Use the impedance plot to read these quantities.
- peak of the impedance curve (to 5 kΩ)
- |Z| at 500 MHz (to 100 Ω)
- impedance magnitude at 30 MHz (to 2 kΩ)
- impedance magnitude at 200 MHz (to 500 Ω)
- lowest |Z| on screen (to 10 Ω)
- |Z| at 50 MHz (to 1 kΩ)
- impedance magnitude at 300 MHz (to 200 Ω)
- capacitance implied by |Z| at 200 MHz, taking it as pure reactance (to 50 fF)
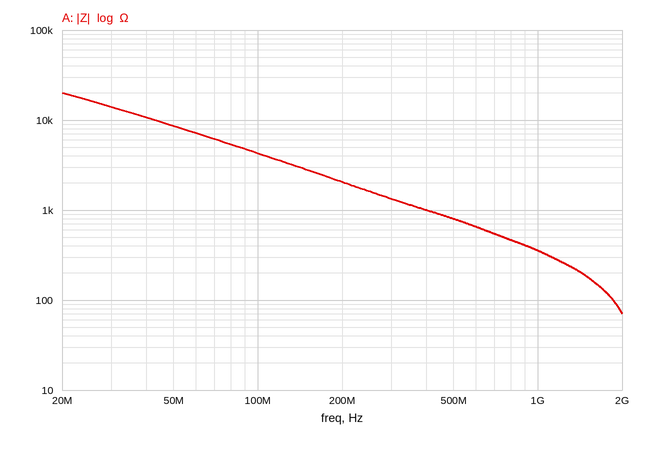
20 kΩ
800 Ω
14 kΩ
2.0 kΩ
70 Ω
9 kΩ
1.4 kΩ
400 fF
